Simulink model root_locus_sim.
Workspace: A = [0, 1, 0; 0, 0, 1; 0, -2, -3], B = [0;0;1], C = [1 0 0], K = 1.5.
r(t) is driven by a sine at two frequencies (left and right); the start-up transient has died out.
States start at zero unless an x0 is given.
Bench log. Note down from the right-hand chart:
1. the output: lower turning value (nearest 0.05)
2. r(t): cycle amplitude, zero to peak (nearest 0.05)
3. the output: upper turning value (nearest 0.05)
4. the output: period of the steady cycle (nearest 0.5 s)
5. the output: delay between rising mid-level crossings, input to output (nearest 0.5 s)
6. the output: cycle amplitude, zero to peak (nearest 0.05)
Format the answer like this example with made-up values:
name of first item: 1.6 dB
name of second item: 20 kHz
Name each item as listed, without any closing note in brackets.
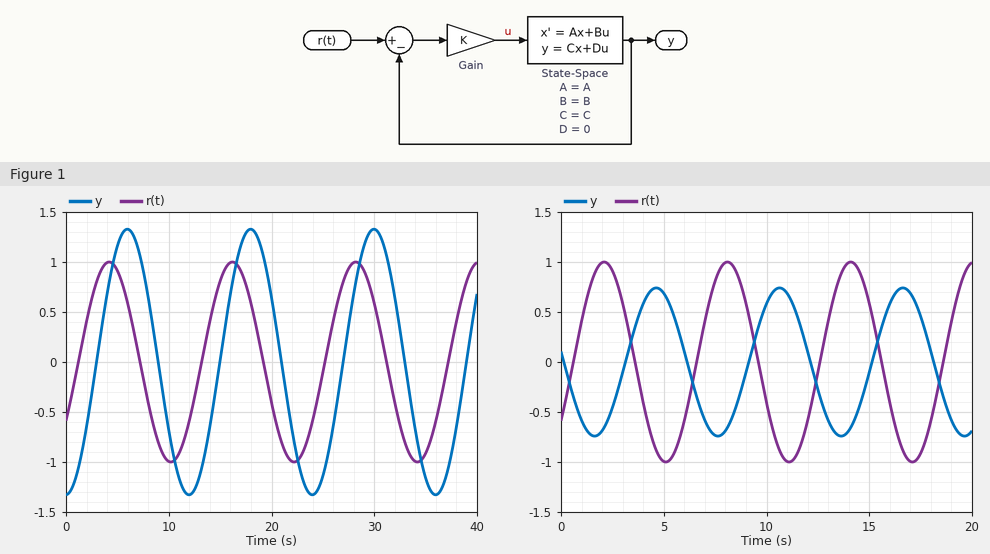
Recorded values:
the output: lower turning value: -0.75
r(t): cycle amplitude, zero to peak: 1.00
the output: upper turning value: 0.75
the output: period of the steady cycle: 6.0 s
the output: delay between rising mid-level crossings, input to output: 2.5 s
the output: cycle amplitude, zero to peak: 0.75
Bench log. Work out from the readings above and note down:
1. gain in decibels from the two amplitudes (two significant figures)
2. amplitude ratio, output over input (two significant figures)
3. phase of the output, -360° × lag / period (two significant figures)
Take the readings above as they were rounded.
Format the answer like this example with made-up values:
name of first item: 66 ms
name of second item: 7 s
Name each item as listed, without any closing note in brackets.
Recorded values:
gain in decibels from the two amplitudes: -2.5 dB
amplitude ratio, output over input: 0.75
phase of the output, -360° × lag / period: -150°
